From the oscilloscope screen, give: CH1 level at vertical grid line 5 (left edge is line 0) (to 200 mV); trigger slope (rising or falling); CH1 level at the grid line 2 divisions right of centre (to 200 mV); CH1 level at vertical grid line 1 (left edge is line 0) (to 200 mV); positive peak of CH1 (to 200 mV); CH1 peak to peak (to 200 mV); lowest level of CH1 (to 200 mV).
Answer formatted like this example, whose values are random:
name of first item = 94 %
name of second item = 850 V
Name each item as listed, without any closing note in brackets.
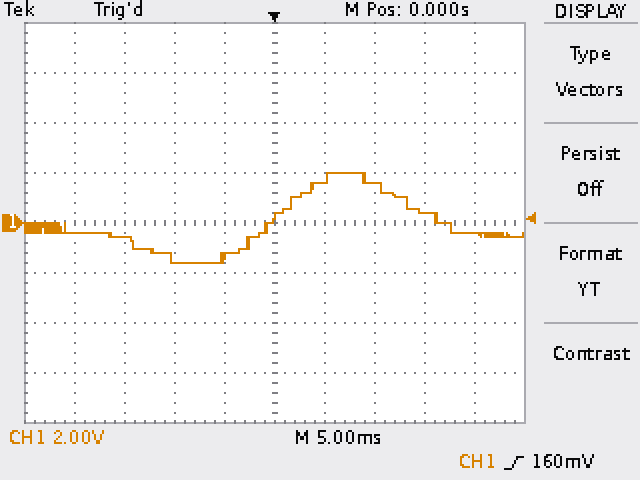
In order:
CH1 level at vertical grid line 5 (left edge is line 0) = 200 mV
trigger slope = rising
CH1 level at the grid line 2 divisions right of centre = 1.6 V
CH1 level at vertical grid line 1 (left edge is line 0) = -400 mV
positive peak of CH1 = 2.0 V
CH1 peak to peak = 3.6 V
lowest level of CH1 = -1.6 V
